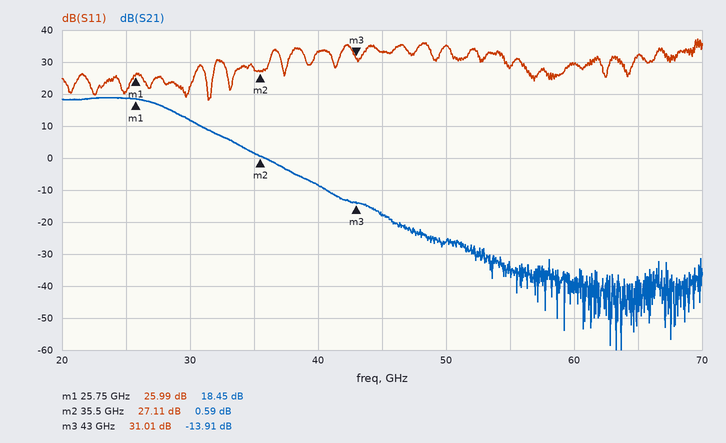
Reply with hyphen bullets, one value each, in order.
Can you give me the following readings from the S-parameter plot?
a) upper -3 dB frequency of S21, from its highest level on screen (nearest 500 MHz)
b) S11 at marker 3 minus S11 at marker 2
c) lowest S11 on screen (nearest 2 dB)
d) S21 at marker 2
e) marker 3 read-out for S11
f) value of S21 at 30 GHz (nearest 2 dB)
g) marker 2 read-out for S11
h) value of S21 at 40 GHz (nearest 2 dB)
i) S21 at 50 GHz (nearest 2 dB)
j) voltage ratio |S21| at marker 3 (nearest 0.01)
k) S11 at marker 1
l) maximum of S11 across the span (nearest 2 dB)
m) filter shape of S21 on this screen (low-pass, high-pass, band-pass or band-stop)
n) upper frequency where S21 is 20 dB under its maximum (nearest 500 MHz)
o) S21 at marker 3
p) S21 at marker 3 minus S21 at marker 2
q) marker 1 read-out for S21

- 28.0 GHz
- 3.90 dB
- 18 dB
- 0.59 dB
- 31.01 dB
- 12 dB
- 27.11 dB
- -8 dB
- -26 dB
- 0.20
- 25.99 dB
- 38 dB
- low-pass
- 36.5 GHz
- -13.91 dB
- -14.50 dB
- 18.45 dB
